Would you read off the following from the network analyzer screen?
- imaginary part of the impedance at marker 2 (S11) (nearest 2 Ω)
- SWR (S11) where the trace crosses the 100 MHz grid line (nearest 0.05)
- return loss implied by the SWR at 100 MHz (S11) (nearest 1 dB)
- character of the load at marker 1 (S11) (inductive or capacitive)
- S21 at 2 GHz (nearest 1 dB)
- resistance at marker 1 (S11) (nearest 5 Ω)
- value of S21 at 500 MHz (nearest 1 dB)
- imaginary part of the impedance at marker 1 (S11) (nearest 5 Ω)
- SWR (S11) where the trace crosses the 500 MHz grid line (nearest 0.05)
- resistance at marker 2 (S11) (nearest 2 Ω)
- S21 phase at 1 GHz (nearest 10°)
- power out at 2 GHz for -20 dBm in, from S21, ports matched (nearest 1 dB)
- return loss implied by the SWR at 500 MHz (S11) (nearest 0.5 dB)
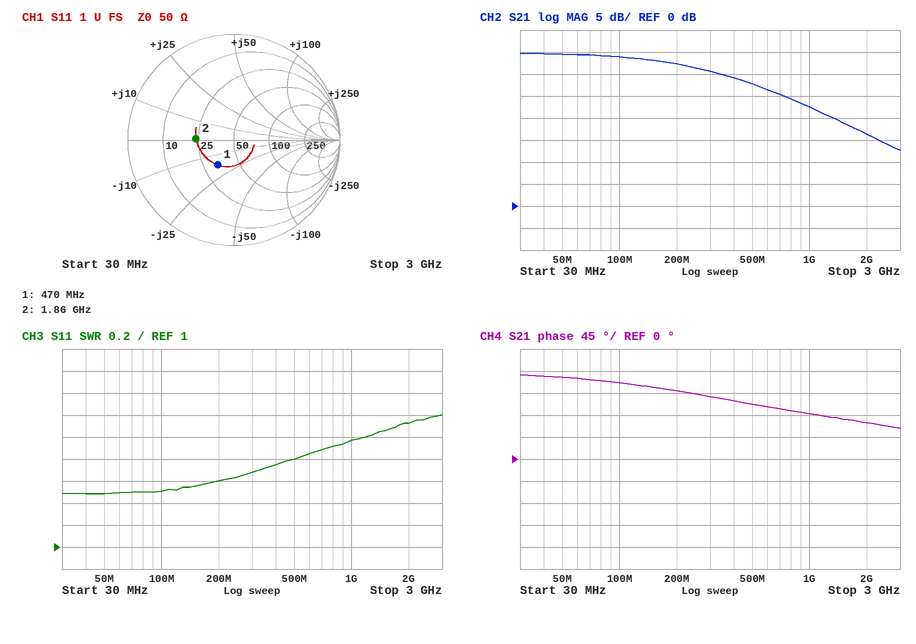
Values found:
0 Ω
1.50
14 dB
capacitive
16 dB
35 Ω
28 dB
-15 Ω
1.80
24 Ω
90°
-4 dBm
11.0 dB
